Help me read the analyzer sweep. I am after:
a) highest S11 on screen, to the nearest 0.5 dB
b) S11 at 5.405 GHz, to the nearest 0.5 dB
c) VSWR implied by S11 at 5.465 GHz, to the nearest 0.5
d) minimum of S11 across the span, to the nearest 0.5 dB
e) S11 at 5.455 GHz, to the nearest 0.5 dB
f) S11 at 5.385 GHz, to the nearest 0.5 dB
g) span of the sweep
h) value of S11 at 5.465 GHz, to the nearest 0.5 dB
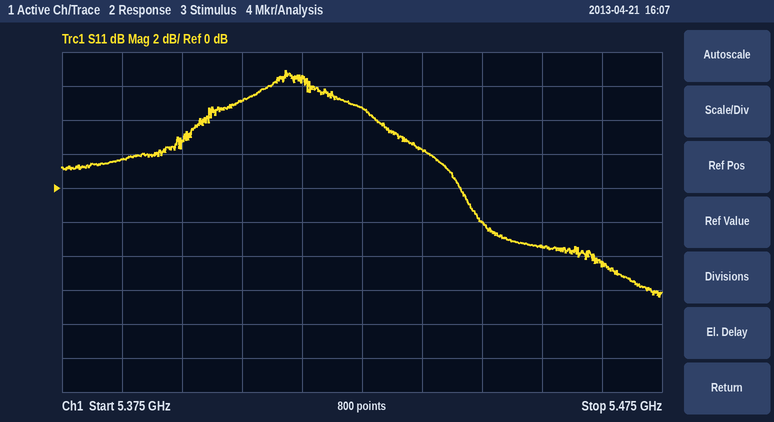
7.0 dB
5.0 dB
4.0
-6.5 dB
-3.5 dB
1.5 dB
100 MHz
-4.5 dB
